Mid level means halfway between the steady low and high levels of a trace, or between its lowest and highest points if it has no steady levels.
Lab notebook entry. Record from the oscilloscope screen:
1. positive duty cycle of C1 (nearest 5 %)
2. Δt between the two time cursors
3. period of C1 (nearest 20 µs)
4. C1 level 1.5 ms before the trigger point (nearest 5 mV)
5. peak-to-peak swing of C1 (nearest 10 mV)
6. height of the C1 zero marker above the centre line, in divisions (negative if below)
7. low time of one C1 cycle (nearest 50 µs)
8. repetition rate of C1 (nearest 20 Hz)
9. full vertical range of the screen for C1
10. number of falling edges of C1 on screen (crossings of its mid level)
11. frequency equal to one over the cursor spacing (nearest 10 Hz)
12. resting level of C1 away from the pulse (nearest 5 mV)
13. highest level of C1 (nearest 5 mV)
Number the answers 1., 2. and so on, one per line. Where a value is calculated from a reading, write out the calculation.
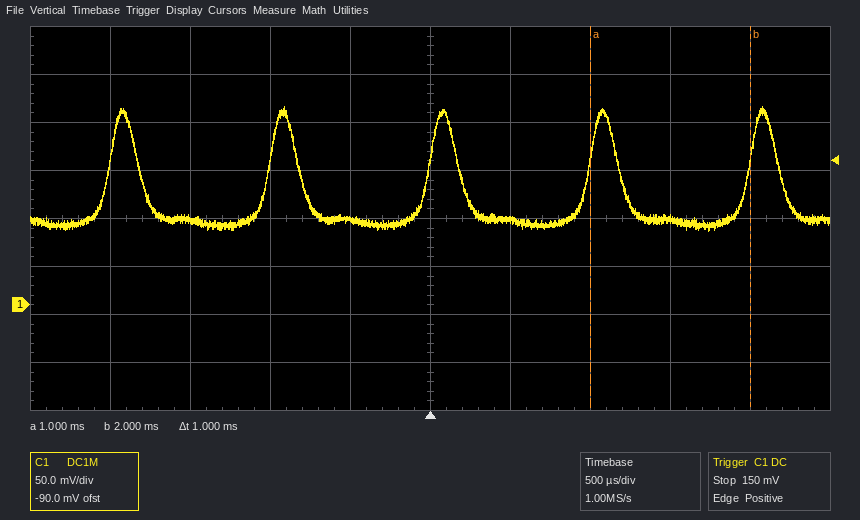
1. 20 %
2. 1 ms
3. 1.00 ms
4. 90 mV
5. 130 mV
6. -1.8 div
7. 800 µs
8. 1 / 1.00 ms ≈ 1.00 kHz
9. 400 mV
10. 5
11. 1 / 1 ms ≈ 1.00 kHz
12. 90 mV
13. 205 mV
